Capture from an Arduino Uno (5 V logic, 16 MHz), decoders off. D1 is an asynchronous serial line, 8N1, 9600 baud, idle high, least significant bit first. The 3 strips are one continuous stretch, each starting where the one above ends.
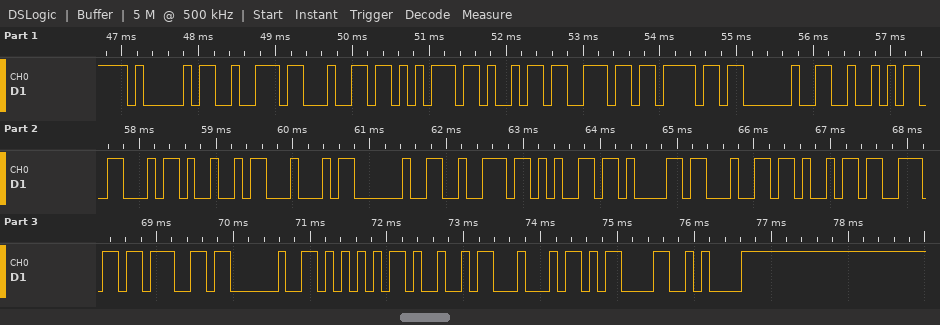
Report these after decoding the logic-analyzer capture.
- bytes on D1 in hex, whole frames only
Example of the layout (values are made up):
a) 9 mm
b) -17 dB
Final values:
a) 41 72 64 75 69 6E 6F 20 52 46 49 44 20 72 65 61 64 69 6E 67 20 55 49 44 0D 0A
